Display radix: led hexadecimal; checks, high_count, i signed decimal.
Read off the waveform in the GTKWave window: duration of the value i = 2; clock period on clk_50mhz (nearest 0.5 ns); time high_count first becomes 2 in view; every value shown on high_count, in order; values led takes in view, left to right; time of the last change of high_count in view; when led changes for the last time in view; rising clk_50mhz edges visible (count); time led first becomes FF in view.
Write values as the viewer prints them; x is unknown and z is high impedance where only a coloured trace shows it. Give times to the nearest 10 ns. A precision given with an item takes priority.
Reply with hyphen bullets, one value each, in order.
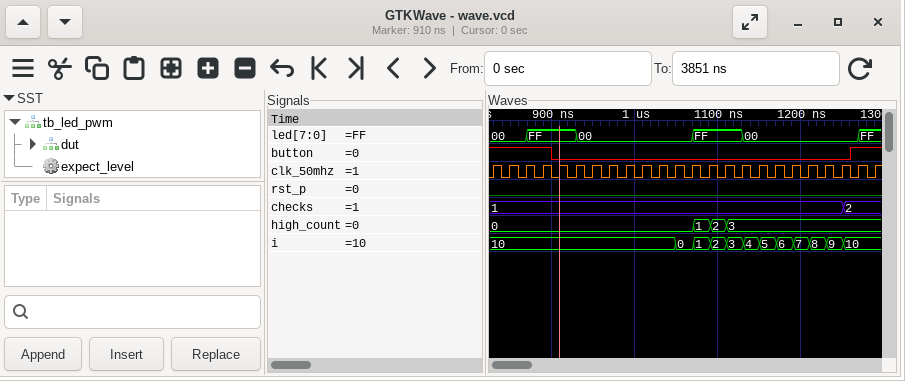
- 20 ns
- 20 ns
- 1090 ns
- 0, 1, 2, 3
- 00, FF, 00, FF, 00, FF
- 1110 ns
- 1270 ns
- 24
- 870 ns
